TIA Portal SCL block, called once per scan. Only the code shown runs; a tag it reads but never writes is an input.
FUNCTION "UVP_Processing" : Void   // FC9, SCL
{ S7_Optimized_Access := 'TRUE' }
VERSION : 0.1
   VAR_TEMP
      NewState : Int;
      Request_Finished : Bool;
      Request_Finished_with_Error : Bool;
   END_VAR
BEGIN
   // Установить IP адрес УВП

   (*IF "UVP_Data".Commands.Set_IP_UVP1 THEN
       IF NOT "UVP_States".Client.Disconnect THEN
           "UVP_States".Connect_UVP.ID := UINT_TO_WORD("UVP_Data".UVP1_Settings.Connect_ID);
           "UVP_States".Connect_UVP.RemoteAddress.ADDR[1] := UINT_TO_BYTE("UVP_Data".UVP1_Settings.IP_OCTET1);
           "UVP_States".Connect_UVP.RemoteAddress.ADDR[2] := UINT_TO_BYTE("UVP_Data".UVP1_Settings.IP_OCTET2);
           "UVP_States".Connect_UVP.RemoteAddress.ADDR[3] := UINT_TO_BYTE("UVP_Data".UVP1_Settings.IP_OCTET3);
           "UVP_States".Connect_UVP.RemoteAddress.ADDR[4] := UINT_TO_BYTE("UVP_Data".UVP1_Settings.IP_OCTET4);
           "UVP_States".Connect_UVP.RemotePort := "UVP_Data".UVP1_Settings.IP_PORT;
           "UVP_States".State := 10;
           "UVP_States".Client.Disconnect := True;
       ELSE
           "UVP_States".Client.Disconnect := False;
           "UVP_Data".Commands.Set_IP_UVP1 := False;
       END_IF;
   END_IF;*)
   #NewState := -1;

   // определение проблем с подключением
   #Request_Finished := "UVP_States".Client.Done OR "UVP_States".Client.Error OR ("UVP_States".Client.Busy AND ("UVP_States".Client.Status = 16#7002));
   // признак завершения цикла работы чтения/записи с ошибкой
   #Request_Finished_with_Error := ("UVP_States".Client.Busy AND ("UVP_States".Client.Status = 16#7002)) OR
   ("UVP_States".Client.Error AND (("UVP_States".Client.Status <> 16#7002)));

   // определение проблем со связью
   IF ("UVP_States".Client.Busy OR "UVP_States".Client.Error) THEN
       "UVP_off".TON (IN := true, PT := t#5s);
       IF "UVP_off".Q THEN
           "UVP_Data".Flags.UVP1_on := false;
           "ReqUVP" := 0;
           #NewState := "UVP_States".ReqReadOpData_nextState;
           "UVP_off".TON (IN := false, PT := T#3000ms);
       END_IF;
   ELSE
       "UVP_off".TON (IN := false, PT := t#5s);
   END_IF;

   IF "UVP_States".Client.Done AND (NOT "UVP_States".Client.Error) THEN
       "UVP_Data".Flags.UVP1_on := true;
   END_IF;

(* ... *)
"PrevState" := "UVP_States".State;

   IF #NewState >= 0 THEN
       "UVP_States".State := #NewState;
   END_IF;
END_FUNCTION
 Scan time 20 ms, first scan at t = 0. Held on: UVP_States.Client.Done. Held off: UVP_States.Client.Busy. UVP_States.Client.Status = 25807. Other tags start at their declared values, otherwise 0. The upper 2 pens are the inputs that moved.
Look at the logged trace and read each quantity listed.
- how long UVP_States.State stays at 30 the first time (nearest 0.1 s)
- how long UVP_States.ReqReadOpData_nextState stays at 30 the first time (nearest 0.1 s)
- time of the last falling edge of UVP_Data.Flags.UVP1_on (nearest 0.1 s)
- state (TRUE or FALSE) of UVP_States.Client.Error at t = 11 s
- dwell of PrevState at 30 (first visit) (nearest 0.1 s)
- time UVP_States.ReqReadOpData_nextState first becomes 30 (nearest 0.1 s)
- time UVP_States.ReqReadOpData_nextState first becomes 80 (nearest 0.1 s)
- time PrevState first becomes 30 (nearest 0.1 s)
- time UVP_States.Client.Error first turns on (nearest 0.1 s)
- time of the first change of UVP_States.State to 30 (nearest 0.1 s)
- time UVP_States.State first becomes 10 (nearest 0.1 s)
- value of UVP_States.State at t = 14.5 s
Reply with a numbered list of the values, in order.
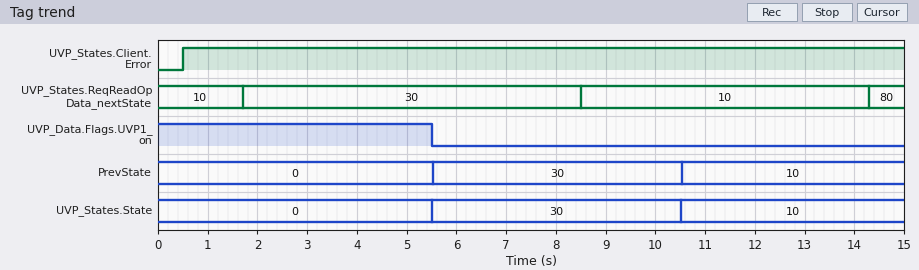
1. 5.0 s
2. 6.8 s
3. 5.5 s
4. TRUE
5. 5.0 s
6. 1.7 s
7. 14.3 s
8. 5.5 s
9. 0.5 s
10. 5.5 s
11. 10.5 s
12. 10
